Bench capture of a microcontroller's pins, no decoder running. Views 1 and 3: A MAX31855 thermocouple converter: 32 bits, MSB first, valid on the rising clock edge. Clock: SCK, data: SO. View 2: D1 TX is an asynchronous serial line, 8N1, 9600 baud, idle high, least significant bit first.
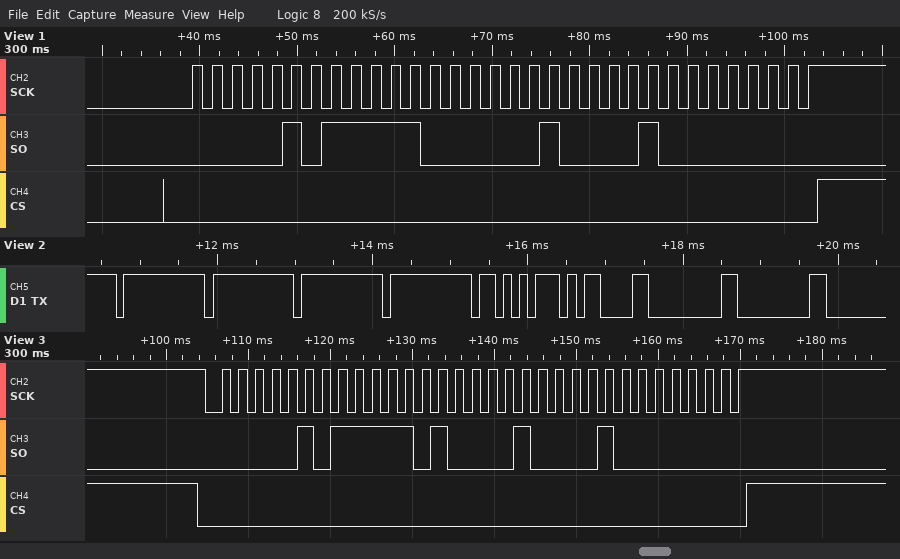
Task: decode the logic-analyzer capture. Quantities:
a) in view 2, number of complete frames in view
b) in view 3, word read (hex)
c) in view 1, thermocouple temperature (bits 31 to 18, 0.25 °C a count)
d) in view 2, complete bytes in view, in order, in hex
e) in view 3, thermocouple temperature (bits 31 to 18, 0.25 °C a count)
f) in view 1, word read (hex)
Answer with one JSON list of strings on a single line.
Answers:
["8", "0x05F42100", "95.00 °C", "FF FF FF FF AB 0D 00 00", "95.25 °C", "0x05F02100"]
